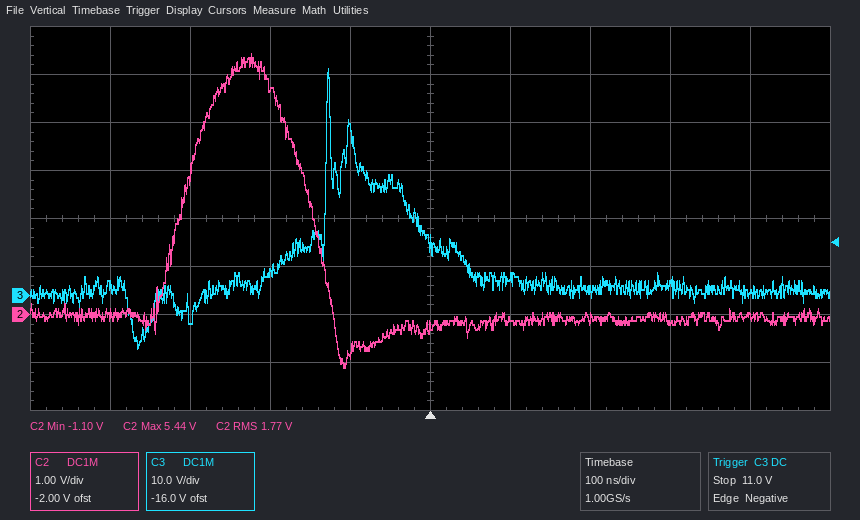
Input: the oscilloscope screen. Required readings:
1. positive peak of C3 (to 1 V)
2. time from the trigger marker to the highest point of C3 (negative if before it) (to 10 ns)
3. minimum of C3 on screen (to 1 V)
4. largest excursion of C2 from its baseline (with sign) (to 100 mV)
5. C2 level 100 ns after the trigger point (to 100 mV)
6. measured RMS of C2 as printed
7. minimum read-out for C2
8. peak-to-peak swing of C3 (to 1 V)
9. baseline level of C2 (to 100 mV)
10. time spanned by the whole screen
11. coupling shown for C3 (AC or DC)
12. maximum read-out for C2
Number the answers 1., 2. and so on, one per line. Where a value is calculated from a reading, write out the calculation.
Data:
1. 47 V
2. -130 ns
3. -11 V
4. +5.5 V
5. -100 mV
6. 1.77 V
7. -1.10 V
8. 47 V − (-11 V) = 58 V
9. -100 mV
10. 1 µs
11. DC
12. 5.44 V
